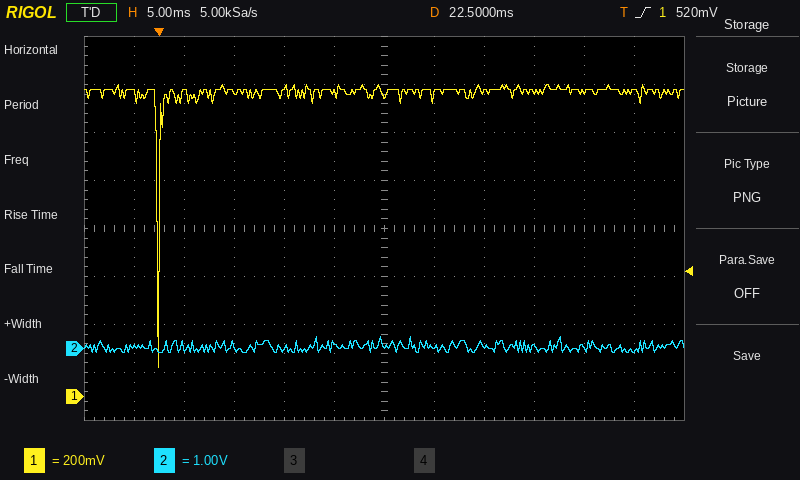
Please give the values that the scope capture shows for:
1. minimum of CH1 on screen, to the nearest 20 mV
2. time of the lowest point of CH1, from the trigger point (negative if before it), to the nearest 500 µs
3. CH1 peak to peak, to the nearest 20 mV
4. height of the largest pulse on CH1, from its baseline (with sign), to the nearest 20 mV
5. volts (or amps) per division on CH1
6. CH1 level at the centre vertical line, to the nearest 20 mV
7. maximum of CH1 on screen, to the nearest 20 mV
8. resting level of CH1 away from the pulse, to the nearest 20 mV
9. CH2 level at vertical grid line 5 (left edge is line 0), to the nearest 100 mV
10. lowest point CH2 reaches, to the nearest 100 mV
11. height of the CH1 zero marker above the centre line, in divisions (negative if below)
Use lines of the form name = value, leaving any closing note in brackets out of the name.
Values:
minimum of CH1 on screen, to the nearest 20 mV = 120 mV
time of the lowest point of CH1, from the trigger point (negative if before it), to the nearest 500 µs = 0.0 ms
CH1 peak to peak, to the nearest 20 mV = 1.18 V
height of the largest pulse on CH1, from its baseline (with sign), to the nearest 20 mV = -1.16 V
volts (or amps) per division on CH1 = 200 mV
CH1 level at the centre vertical line, to the nearest 20 mV = 1.26 V
maximum of CH1 on screen, to the nearest 20 mV = 1.30 V
resting level of CH1 away from the pulse, to the nearest 20 mV = 1.28 V
CH2 level at vertical grid line 5 (left edge is line 0), to the nearest 100 mV = 100 mV
lowest point CH2 reaches, to the nearest 100 mV = -100 mV
height of the CH1 zero marker above the centre line, in divisions = -3.5 div
